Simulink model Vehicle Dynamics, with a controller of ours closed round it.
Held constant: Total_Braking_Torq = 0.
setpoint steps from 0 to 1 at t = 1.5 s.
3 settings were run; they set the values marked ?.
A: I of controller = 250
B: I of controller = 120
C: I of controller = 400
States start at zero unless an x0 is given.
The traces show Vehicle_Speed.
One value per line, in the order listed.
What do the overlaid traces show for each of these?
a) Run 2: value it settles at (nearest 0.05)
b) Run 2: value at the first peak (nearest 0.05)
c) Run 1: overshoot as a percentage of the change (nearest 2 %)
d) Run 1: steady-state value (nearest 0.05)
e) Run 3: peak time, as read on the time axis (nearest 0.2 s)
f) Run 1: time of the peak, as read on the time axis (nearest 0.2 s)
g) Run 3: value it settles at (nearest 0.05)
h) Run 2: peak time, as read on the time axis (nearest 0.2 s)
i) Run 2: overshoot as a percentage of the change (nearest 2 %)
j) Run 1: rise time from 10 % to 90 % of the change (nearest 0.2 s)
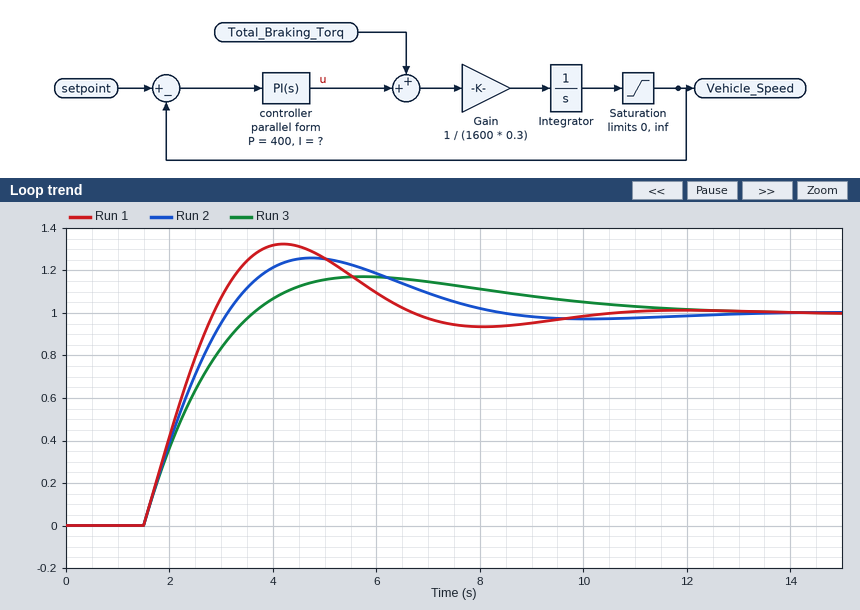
1.00
1.25
32 %
1.00
5.8 s
4.2 s
1.00
4.8 s
26 %
1.0 s
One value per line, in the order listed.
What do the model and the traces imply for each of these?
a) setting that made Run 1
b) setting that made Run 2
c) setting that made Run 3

C
A
B
